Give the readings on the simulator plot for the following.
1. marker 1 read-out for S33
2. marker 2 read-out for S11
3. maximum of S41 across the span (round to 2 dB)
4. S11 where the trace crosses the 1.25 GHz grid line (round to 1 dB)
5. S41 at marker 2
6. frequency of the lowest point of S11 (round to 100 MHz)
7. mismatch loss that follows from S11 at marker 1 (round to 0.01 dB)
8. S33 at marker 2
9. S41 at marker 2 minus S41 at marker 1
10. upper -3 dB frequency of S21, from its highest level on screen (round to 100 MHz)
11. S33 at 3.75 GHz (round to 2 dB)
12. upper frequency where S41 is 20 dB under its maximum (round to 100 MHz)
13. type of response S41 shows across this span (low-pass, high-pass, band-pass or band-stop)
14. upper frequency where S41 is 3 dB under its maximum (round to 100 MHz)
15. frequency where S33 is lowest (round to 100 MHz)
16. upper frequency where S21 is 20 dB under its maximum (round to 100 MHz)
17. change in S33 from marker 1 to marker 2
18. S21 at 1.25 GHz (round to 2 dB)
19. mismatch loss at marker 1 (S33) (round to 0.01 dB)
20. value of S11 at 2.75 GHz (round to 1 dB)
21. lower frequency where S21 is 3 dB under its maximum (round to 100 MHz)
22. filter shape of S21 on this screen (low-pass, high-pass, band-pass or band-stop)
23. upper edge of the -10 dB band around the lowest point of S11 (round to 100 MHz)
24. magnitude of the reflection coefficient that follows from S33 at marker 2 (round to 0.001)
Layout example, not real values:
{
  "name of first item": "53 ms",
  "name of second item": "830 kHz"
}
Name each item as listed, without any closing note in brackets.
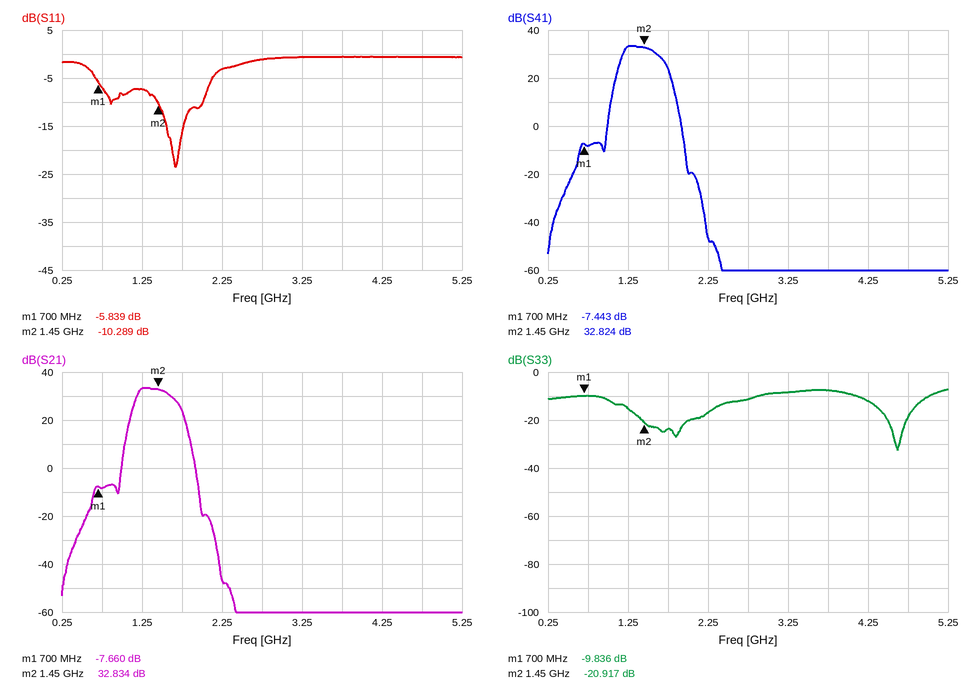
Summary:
{
  "marker 1 read-out for S33": "-9.836 dB",
  "marker 2 read-out for S11": "-10.289 dB",
  "maximum of S41 across the span": "34 dB",
  "S11 where the trace crosses the 1.25 GHz grid line": "-7 dB",
  "S41 at marker 2": "32.824 dB",
  "frequency of the lowest point of S11": "1.7 GHz",
  "mismatch loss that follows from S11 at marker 1": "1.31 dB",
  "S33 at marker 2": "-20.917 dB",
  "S41 at marker 2 minus S41 at marker 1": "40.267 dB",
  "upper -3 dB frequency of S21, from its highest level on screen": "1.6 GHz",
  "S33 at 3.75 GHz": "-8 dB",
  "upper frequency where S41 is 20 dB under its maximum": "1.8 GHz",
  "type of response S41 shows across this span": "band-pass",
  "upper frequency where S41 is 3 dB under its maximum": "1.6 GHz",
  "frequency where S33 is lowest": "4.6 GHz",
  "upper frequency where S21 is 20 dB under its maximum": "1.8 GHz",
  "change in S33 from marker 1 to marker 2": "-11.081 dB",
  "S21 at 1.25 GHz": "34 dB",
  "mismatch loss at marker 1 (S33)": "0.48 dB",
  "value of S11 at 2.75 GHz": "-1 dB",
  "lower frequency where S21 is 3 dB under its maximum": "1.2 GHz",
  "filter shape of S21 on this screen": "band-pass",
  "upper edge of the -10 dB band around the lowest point of S11": "2.0 GHz",
  "magnitude of the reflection coefficient that follows from S33 at marker 2": "0.090"
}
